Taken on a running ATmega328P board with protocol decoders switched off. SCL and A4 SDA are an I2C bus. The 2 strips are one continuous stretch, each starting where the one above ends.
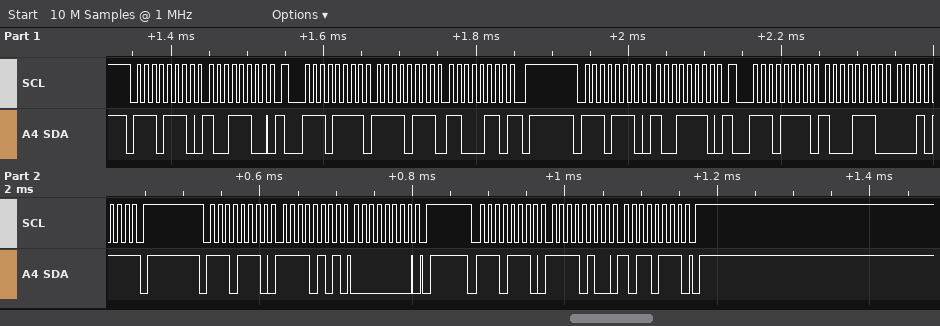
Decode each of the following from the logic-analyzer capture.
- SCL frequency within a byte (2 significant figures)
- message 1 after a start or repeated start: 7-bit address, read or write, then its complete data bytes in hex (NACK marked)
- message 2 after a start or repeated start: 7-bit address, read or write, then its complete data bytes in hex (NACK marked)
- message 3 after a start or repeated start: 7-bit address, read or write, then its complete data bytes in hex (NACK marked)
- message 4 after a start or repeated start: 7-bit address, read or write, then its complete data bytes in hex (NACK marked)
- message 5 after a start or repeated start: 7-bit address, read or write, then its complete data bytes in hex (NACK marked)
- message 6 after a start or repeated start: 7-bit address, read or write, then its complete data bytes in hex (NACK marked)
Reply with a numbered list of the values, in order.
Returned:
1. 100 kHz
2. 0x77 write: 9C
3. 0x77 read: F7 C6 NACK
4. 0x77 write: 9E
5. 0x77 read: 8E 17 NACK
6. 0x77 write: F5 00
7. 0x77 write: F4 B7
